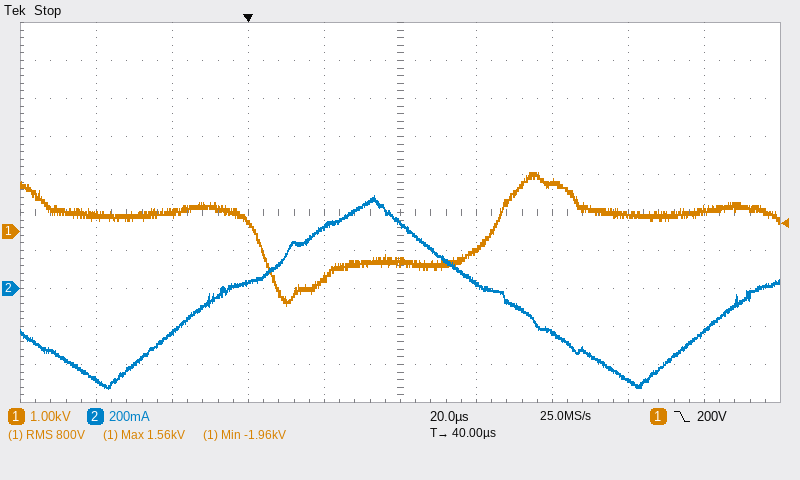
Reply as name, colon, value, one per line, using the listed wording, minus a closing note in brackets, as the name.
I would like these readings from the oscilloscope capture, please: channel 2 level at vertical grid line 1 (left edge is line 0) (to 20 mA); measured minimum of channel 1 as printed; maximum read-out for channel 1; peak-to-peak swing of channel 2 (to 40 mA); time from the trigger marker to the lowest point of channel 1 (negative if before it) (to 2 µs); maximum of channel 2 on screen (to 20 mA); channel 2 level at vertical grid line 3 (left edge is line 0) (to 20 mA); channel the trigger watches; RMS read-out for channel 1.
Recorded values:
channel 2 level at vertical grid line 1 (left edge is line 0): -480 mA
measured minimum of channel 1 as printed: -1.96 kV
maximum read-out for channel 1: 1.56 kV
peak-to-peak swing of channel 2: 1.00 A
time from the trigger marker to the lowest point of channel 1 (negative if before it): +10 µs
maximum of channel 2 on screen: 480 mA
channel 2 level at vertical grid line 3 (left edge is line 0): 40 mA
channel the trigger watches: channel 1
RMS read-out for channel 1: 800 V
